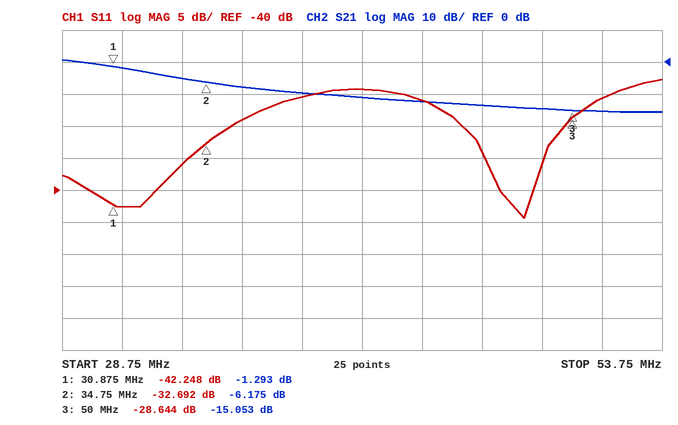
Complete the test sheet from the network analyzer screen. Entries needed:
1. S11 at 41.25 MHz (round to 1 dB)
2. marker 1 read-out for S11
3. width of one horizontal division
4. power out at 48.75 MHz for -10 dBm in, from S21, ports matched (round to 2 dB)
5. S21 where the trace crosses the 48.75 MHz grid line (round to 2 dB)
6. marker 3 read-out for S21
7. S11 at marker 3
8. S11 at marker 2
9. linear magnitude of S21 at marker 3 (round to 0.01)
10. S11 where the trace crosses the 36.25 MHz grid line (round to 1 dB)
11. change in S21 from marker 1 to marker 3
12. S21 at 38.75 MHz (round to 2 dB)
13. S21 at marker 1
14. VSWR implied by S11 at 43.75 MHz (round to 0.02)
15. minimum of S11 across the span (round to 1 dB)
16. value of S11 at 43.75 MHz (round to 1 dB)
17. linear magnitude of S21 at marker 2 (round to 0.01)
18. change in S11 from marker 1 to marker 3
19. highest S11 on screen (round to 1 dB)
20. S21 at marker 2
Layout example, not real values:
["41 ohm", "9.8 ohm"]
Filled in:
["-24 dB", "-42.248 dB", "2.5 MHz", "-24 dBm", "-14 dB", "-15.053 dB", "-28.644 dB", "-32.692 dB", "0.18", "-29 dB", "-13.760 dB", "-10 dB", "-1.293 dB", "1.10", "-44 dB", "-26 dB", "0.49", "13.604 dB", "-23 dB", "-6.175 dB"]
